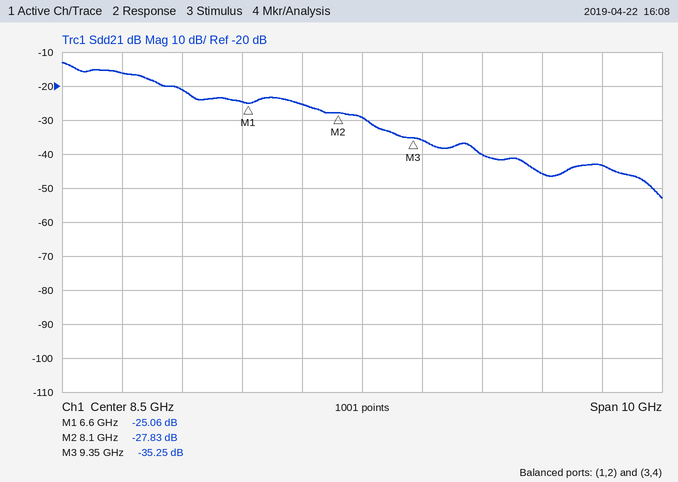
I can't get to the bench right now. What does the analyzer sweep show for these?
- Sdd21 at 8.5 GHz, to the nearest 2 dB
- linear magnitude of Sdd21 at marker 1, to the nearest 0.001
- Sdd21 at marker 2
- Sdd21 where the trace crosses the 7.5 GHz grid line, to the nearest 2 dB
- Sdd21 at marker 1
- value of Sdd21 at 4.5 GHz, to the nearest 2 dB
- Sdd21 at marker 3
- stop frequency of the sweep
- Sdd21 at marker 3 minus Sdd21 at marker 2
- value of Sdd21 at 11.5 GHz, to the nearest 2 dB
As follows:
-30 dB
0.056
-27.83 dB
-26 dB
-25.06 dB
-16 dB
-35.25 dB
13.5 GHz
-7.42 dB
-46 dB
